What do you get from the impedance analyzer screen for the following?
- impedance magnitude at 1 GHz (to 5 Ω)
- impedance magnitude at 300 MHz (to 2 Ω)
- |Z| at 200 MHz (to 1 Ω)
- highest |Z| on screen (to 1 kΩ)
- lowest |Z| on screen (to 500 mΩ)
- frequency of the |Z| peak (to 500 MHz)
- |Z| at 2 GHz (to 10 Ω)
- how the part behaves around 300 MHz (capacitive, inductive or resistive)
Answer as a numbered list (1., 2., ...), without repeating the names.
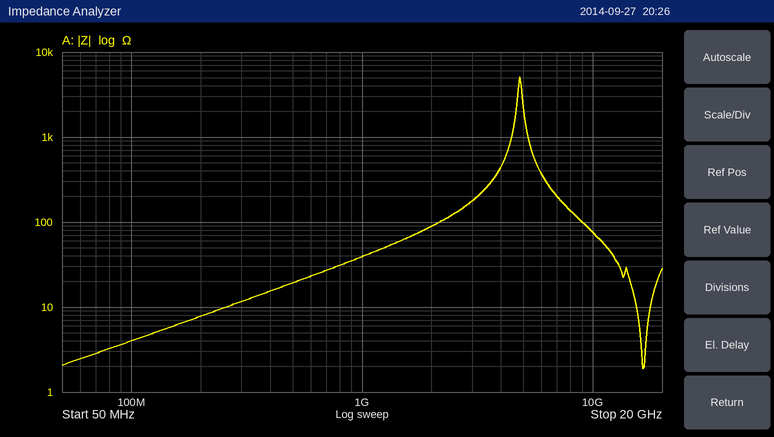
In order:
1. 40 Ω
2. 12 Ω
3. 8 Ω
4. 5 kΩ
5. 2.0 Ω
6. 5.0 GHz
7. 90 Ω
8. inductive
